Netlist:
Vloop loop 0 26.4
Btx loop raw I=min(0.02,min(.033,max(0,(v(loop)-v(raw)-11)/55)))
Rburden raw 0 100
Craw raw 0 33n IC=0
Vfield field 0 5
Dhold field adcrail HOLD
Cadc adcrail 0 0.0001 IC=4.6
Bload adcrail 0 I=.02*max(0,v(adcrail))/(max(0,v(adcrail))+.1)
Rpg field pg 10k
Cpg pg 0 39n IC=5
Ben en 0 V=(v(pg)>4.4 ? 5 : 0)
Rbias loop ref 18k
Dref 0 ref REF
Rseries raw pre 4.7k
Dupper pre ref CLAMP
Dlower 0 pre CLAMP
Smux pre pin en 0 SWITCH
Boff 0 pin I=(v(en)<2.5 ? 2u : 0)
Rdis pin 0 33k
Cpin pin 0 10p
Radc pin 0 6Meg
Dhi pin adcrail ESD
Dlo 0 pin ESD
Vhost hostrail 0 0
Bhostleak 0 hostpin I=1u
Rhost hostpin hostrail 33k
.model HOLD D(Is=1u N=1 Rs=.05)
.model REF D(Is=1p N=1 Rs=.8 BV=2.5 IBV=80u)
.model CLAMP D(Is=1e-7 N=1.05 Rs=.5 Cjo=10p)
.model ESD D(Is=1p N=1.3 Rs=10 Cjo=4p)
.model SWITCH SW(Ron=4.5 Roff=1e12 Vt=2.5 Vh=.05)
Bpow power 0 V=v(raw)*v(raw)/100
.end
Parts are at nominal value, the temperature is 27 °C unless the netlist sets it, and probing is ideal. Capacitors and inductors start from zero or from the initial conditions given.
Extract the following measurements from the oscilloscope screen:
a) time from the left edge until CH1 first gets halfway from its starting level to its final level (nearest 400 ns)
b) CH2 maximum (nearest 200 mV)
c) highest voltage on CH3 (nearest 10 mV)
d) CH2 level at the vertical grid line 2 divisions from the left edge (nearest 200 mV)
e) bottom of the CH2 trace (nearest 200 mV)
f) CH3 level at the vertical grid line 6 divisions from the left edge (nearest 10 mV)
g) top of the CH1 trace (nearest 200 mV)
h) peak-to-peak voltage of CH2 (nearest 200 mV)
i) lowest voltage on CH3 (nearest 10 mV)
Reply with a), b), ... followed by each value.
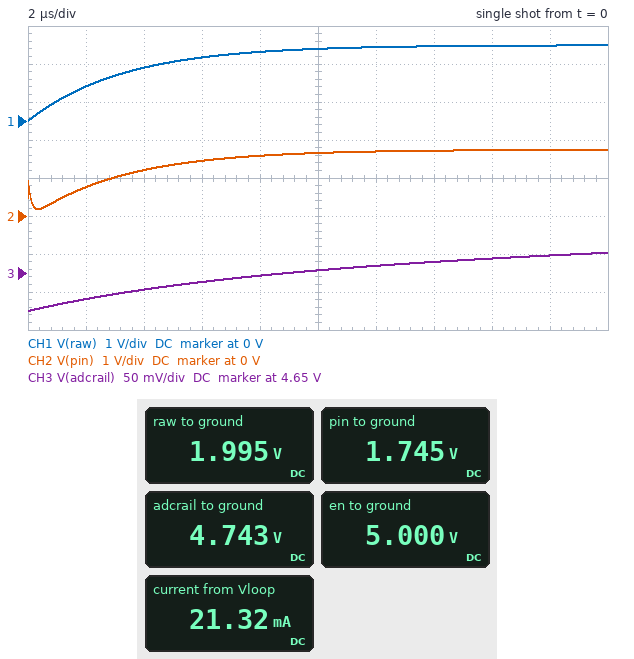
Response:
a) 2.4 µs
b) 1.8 V
c) 4.68 V
d) 1.2 V
e) 200 mV
f) 4.66 V
g) 2.0 V
h) 1.6 V
i) 4.60 V
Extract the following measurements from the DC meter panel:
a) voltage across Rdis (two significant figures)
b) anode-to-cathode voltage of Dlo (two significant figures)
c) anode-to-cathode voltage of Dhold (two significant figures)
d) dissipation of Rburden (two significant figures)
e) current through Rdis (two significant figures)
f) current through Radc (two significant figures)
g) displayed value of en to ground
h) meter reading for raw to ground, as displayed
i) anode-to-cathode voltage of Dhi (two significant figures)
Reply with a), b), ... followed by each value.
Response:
a) 1.7 V
b) -1.7 V
c) 260 mV
d) 40 mW
e) 53 µA
f) 290 nA
g) 5.000 V
h) 1.995 V
i) -3.0 V
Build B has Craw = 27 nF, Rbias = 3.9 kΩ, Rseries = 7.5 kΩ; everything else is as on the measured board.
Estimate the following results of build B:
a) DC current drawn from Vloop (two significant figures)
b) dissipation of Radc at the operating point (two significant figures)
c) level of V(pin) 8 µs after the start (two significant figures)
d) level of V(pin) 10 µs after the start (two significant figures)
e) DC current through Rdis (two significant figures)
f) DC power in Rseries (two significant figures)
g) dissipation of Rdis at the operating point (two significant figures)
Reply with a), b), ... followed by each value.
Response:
a) 26 mA
b) 440 nW
c) 1.5 V
d) 1.6 V
e) 49 µA
f) 18 µW
g) 80 µW
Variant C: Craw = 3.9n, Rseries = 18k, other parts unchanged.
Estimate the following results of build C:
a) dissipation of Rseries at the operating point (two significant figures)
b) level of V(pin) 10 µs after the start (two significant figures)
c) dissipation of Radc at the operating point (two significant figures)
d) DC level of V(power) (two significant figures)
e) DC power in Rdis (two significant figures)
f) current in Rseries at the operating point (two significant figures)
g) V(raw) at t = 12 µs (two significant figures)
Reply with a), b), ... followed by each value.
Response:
a) 28 µW
b) 1.3 V
c) 280 nW
d) 40 mV
e) 50 µW
f) 39 µA
g) 2.0 V
